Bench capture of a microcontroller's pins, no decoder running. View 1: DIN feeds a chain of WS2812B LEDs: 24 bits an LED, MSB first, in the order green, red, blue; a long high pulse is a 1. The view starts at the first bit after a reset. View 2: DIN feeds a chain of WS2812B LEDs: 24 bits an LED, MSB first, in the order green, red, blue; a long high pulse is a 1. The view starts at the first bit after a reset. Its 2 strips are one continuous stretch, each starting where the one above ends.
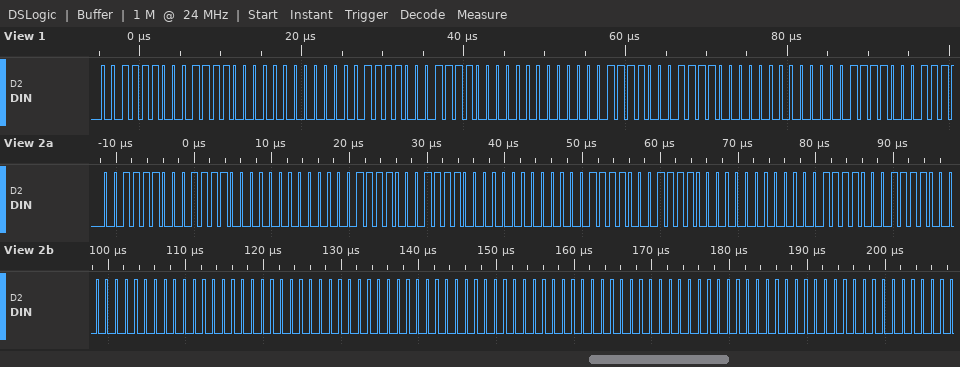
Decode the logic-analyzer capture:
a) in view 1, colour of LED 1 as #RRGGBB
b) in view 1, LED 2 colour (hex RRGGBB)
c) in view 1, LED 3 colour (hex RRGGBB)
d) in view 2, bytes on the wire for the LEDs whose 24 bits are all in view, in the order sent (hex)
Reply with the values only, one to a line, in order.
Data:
#783C00
#783C00
#783C00
3C 78 00 3C 78 00 3C 78 00 3C 78 00 00 00 00 00 00 00 00 00 00
